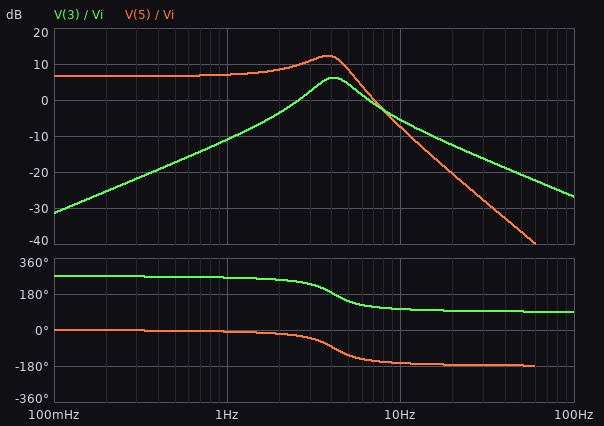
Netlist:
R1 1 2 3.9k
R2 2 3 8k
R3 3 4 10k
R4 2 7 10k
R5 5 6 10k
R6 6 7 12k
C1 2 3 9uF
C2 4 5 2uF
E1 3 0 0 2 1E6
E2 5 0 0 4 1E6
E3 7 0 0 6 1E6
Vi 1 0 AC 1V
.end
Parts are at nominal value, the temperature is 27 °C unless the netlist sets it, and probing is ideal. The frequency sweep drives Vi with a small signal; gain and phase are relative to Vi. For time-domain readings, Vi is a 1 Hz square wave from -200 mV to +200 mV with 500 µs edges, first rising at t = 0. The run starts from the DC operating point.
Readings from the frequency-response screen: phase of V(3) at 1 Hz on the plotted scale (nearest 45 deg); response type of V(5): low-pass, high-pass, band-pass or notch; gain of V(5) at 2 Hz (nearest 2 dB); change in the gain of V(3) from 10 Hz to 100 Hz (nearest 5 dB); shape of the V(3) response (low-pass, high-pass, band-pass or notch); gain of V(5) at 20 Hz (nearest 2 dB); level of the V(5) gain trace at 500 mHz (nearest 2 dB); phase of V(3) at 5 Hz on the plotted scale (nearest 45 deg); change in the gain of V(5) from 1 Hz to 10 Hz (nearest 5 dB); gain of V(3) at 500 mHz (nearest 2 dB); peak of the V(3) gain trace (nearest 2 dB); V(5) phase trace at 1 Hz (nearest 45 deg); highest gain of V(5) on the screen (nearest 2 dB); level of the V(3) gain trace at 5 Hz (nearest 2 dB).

270 deg
low-pass
8 dB
-20 dB
band-pass
-20 dB
6 dB
135 deg
-15 dB
-18 dB
6 dB
0 deg
12 dB
4 dB
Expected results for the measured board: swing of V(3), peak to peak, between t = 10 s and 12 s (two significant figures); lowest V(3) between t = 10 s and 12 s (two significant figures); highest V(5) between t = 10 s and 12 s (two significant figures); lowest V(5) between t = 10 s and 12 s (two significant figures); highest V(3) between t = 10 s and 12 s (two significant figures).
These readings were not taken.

600 mV
-300 mV
770 mV
-770 mV
300 mV
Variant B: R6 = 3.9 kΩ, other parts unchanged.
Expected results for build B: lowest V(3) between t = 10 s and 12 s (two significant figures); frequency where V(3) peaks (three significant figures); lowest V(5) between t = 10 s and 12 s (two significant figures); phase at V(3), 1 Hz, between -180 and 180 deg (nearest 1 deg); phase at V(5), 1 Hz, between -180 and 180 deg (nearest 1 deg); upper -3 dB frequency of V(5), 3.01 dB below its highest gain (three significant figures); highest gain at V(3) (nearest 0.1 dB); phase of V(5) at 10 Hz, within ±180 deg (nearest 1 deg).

-420 mV
2.34 Hz
-1.8 V
-116 deg
-26 deg
2.76 Hz
6.2 dB
-167 deg
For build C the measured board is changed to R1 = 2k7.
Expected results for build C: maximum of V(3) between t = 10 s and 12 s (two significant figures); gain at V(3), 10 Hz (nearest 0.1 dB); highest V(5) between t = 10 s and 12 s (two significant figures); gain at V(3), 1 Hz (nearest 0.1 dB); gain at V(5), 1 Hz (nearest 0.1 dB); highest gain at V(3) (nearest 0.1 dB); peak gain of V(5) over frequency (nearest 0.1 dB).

430 mV
-2.4 dB
1.1 V
-7.8 dB
10.2 dB
9.4 dB
15.5 dB
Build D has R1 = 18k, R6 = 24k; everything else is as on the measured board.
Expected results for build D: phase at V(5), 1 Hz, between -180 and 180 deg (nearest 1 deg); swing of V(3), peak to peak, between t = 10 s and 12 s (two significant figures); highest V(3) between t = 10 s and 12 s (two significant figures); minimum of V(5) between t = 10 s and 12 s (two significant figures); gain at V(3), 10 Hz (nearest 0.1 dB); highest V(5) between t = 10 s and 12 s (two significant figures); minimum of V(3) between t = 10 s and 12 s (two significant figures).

-4 deg
100 mV
51 mV
-96 mV
-17.0 dB
96 mV
-51 mV
